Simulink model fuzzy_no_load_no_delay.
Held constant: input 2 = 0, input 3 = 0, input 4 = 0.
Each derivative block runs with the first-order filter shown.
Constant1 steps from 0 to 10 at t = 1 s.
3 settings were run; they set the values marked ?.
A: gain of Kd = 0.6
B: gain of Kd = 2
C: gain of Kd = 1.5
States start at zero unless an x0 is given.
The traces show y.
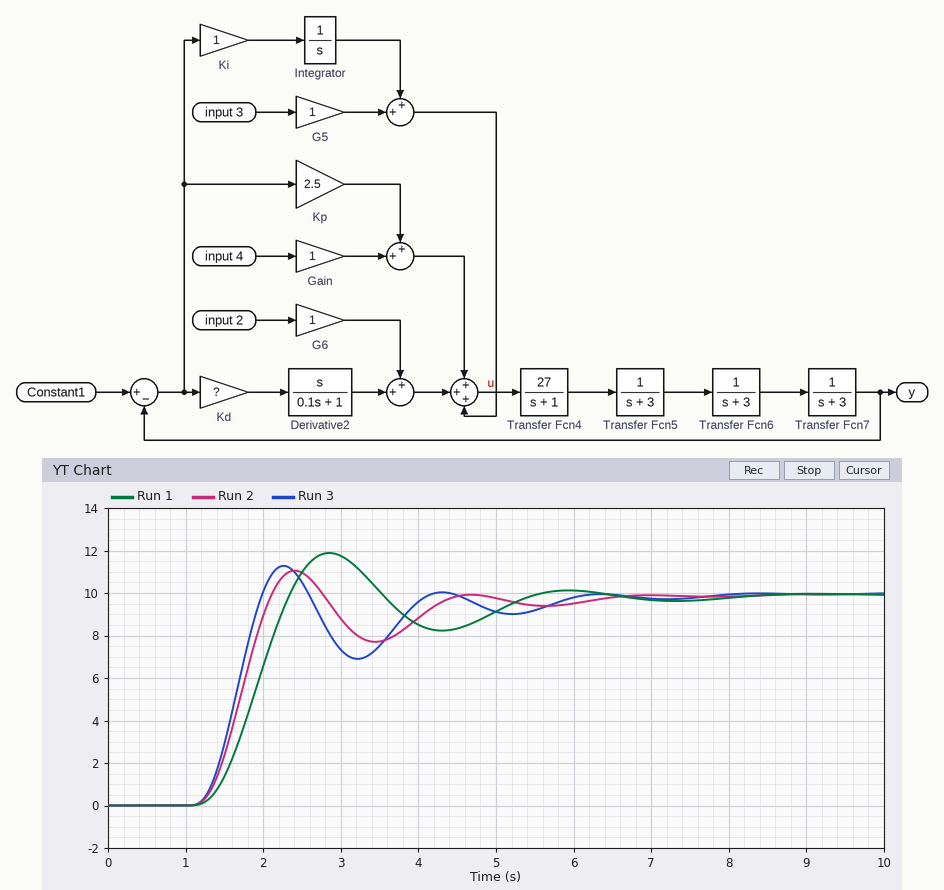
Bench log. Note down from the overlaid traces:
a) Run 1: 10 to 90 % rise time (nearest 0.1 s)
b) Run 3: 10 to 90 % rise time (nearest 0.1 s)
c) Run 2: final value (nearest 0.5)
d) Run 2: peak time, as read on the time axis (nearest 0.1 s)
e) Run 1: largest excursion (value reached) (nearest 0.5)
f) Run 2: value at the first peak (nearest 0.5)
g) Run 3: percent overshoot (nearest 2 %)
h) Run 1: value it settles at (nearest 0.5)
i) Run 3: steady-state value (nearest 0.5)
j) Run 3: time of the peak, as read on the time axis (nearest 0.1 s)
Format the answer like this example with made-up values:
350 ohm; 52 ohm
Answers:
0.8 s; 0.6 s; 10.0; 2.4 s; 12.0; 11.0; 12 %; 10.0; 10.0; 2.3 s
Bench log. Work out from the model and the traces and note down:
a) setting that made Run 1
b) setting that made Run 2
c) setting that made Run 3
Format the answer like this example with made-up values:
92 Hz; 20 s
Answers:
A; C; B
